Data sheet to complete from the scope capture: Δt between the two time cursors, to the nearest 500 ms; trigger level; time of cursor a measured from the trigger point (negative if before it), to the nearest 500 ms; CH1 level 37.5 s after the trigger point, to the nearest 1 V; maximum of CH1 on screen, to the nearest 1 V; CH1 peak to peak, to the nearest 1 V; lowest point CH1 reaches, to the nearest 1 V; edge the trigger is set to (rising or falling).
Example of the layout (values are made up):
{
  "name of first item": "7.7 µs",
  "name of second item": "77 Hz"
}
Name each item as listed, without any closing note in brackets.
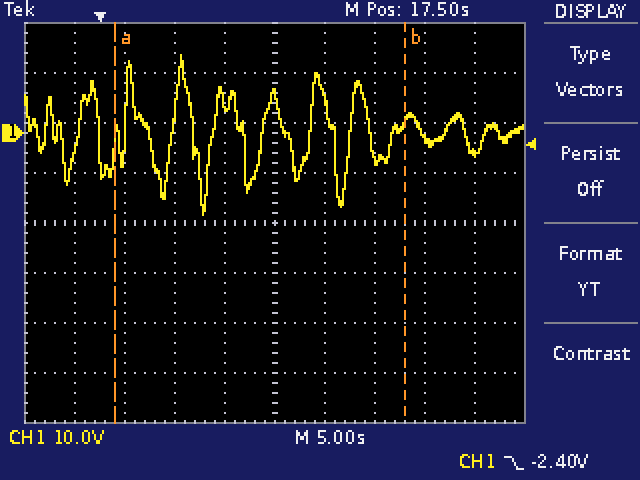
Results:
{
  "Δt between the two time cursors, to the nearest 500 ms": "29.0 s",
  "trigger level": "-2.40 V",
  "time of cursor a measured from the trigger point (negative if before it), to the nearest 500 ms": "+1.5 s",
  "CH1 level 37.5 s after the trigger point, to the nearest 1 V": "-4 V",
  "maximum of CH1 on screen, to the nearest 1 V": "16 V",
  "CH1 peak to peak, to the nearest 1 V": "32 V",
  "lowest point CH1 reaches, to the nearest 1 V": "-16 V",
  "edge the trigger is set to": "falling"
}
